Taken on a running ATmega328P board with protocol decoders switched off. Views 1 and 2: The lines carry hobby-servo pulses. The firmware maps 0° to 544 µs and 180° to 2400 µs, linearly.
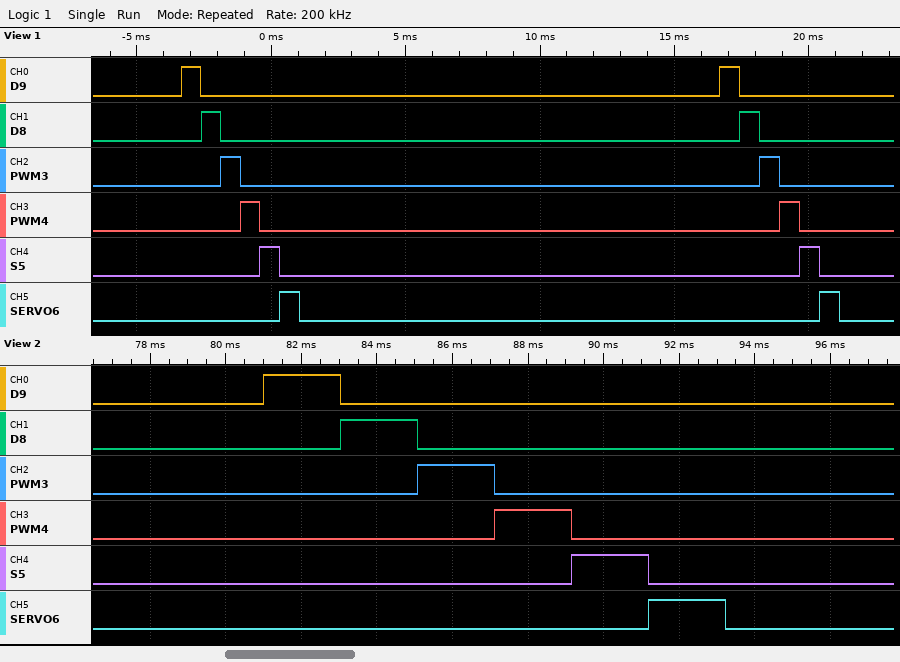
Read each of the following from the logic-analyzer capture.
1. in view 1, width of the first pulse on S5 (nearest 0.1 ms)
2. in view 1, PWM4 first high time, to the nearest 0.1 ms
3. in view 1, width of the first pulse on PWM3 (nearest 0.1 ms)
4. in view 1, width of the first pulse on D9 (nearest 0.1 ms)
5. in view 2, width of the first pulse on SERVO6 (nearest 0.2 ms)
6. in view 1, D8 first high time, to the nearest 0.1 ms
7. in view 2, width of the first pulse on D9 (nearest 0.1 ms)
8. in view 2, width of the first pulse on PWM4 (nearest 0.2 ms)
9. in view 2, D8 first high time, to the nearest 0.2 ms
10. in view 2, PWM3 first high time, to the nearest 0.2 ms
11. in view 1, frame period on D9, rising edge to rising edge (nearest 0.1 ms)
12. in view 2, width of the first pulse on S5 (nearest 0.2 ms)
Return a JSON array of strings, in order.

["0.7 ms", "0.7 ms", "0.7 ms", "0.7 ms", "2.0 ms", "0.7 ms", "2.0 ms", "2.0 ms", "2.0 ms", "2.0 ms", "20.0 ms", "2.0 ms"]
